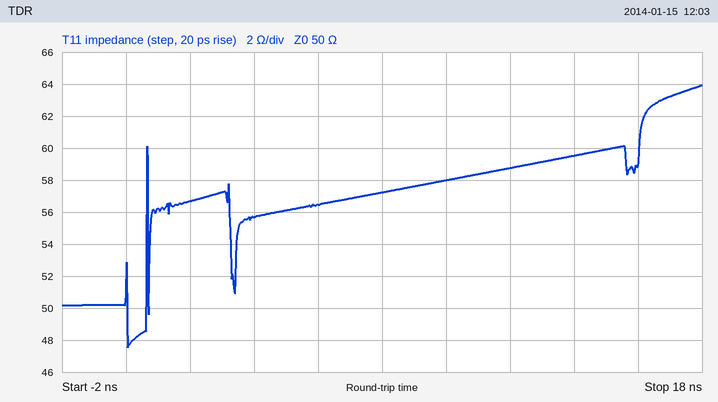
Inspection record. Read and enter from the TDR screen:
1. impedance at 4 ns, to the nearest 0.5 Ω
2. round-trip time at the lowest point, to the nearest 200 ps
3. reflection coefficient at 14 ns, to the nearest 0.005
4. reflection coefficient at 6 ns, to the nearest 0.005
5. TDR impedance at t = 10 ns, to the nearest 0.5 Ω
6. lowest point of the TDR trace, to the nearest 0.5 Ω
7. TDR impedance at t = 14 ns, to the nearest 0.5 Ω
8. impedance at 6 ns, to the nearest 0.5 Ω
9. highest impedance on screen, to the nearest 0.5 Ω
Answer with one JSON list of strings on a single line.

["55.5 Ω", "0.0 ns", "+0.085", "+0.060", "58.0 Ω", "47.5 Ω", "59.5 Ω", "56.5 Ω", "64.0 Ω"]
